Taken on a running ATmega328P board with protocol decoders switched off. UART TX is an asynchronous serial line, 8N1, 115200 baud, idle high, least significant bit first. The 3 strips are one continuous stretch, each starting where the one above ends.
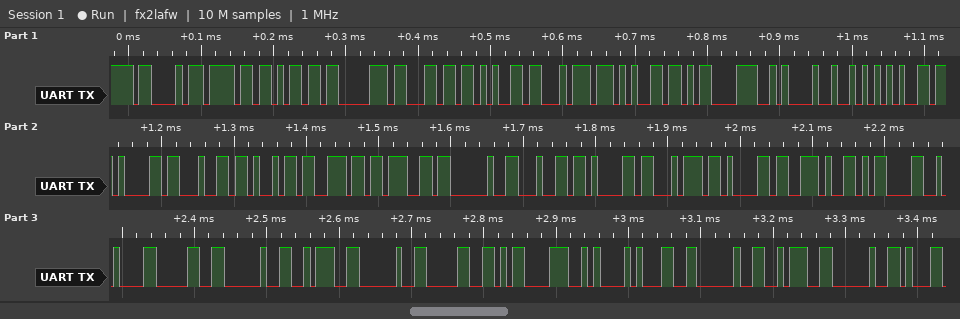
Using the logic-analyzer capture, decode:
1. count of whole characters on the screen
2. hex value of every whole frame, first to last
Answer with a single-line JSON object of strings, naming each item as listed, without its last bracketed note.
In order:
{"count of whole characters on the screen": "36", "hex value of every whole frame, first to last": "43 6F 6D 70 6C 65 74 65 0D 0A 52 65 61 64 69 6E 67 20 64 61 74 61 2E 0D 0A 30 20 3A 20 30 0D 0A 31 20 3A 20"}
